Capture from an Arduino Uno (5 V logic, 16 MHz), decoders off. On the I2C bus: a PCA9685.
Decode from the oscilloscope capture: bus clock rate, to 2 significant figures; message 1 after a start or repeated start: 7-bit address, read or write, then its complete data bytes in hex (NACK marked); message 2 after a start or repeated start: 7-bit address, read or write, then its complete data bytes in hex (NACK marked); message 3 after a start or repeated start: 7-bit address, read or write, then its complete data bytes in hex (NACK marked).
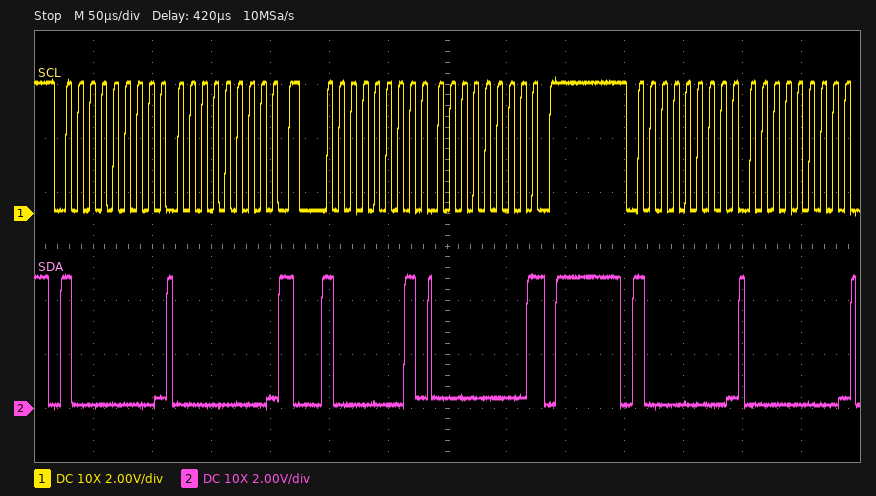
100 kHz
0x40 write: 00
0x40 read: 00 NACK
0x40 write: 00
